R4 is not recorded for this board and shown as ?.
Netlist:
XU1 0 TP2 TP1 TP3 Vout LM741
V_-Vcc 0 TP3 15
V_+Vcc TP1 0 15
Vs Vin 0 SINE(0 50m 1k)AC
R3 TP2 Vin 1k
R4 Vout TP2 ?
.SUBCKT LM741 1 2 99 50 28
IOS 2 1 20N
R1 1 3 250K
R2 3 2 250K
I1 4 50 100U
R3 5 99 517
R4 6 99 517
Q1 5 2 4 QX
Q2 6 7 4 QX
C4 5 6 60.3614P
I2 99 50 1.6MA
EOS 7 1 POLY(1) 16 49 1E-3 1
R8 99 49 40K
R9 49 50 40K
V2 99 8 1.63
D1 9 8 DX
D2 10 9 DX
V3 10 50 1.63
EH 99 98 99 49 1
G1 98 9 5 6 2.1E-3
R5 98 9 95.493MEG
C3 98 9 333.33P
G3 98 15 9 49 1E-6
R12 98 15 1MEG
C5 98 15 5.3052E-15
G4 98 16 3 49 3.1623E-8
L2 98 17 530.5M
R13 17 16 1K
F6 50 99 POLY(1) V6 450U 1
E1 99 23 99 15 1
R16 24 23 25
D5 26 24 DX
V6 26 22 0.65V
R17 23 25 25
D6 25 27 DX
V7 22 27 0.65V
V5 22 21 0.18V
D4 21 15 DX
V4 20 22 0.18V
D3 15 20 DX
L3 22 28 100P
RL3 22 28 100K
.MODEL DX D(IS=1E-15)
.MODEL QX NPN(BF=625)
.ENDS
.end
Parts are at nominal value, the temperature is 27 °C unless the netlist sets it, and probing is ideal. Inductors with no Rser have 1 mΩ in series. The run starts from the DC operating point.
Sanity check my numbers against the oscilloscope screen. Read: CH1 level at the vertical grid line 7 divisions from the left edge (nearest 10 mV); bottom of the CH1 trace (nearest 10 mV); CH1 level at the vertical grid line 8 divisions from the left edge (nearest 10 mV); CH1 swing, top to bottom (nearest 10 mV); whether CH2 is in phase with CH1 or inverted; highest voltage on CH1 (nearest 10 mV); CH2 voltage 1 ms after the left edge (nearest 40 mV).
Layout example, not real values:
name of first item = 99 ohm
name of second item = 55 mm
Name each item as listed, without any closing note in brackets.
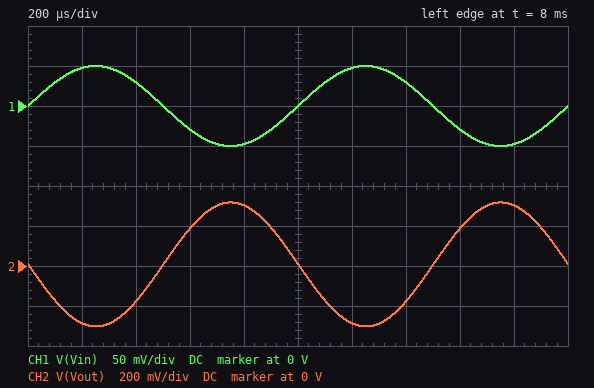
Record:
CH1 level at the vertical grid line 7 divisions from the left edge = 30 mV
bottom of the CH1 trace = -50 mV
CH1 level at the vertical grid line 8 divisions from the left edge = -30 mV
CH1 swing, top to bottom = 100 mV
whether CH2 is in phase with CH1 or inverted = inverted
highest voltage on CH1 = 50 mV
CH2 voltage 1 ms after the left edge = 0 V
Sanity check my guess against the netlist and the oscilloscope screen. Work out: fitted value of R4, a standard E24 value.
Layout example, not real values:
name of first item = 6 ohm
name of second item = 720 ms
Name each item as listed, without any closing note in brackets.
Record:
fitted value of R4, a standard E24 value = 6.2 kΩ
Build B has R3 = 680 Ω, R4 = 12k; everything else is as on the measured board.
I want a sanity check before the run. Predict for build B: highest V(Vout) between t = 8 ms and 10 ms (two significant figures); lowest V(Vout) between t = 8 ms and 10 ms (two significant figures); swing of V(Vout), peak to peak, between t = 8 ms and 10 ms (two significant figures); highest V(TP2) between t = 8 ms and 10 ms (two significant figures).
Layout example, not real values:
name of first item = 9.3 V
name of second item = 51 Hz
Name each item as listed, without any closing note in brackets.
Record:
highest V(Vout) between t = 8 ms and 10 ms = 900 mV
lowest V(Vout) between t = 8 ms and 10 ms = -860 mV
swing of V(Vout), peak to peak, between t = 8 ms and 10 ms = 1.8 V
highest V(TP2) between t = 8 ms and 10 ms = 1.9 mV
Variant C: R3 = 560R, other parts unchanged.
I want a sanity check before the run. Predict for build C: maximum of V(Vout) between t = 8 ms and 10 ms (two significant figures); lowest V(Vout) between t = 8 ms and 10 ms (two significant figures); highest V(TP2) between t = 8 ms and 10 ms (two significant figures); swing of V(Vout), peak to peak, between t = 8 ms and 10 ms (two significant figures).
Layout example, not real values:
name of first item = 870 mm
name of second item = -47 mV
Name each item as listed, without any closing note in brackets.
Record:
maximum of V(Vout) between t = 8 ms and 10 ms = 570 mV
lowest V(Vout) between t = 8 ms and 10 ms = -540 mV
highest V(TP2) between t = 8 ms and 10 ms = 1.6 mV
swing of V(Vout), peak to peak, between t = 8 ms and 10 ms = 1.1 V
